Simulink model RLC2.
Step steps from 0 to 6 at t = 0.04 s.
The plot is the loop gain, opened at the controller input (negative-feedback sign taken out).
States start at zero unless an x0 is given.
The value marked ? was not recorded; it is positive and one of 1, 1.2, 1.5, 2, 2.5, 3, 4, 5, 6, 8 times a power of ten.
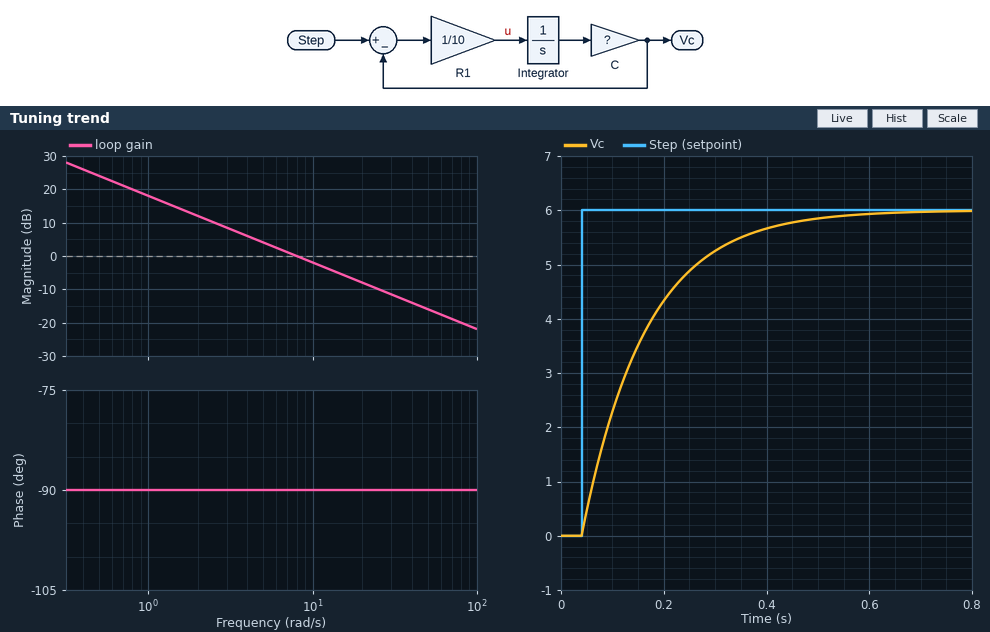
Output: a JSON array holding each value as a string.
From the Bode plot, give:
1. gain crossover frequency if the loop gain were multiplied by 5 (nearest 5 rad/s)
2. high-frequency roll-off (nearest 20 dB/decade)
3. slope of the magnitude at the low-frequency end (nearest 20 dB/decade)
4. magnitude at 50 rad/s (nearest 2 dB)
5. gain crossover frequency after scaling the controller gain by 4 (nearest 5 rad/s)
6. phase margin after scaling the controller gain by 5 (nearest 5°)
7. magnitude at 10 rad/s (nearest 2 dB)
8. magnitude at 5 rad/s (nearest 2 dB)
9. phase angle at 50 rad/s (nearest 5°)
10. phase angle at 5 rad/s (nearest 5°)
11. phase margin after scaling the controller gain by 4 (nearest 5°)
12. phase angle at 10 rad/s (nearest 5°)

["40 rad/s", "-20 dB/decade", "-20 dB/decade", "-16 dB", "30 rad/s", "90°", "-2 dB", "4 dB", "-90°", "-90°", "90°", "-90°"]
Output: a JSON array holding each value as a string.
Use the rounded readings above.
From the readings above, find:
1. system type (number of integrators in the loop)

["1"]
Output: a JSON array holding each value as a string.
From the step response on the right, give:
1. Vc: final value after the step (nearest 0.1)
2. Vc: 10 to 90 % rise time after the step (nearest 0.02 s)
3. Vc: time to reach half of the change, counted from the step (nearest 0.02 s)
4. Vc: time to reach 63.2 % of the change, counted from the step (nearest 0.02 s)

["6.0", "0.28 s", "0.08 s", "0.12 s"]
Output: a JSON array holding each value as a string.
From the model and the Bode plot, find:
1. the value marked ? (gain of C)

["80"]
